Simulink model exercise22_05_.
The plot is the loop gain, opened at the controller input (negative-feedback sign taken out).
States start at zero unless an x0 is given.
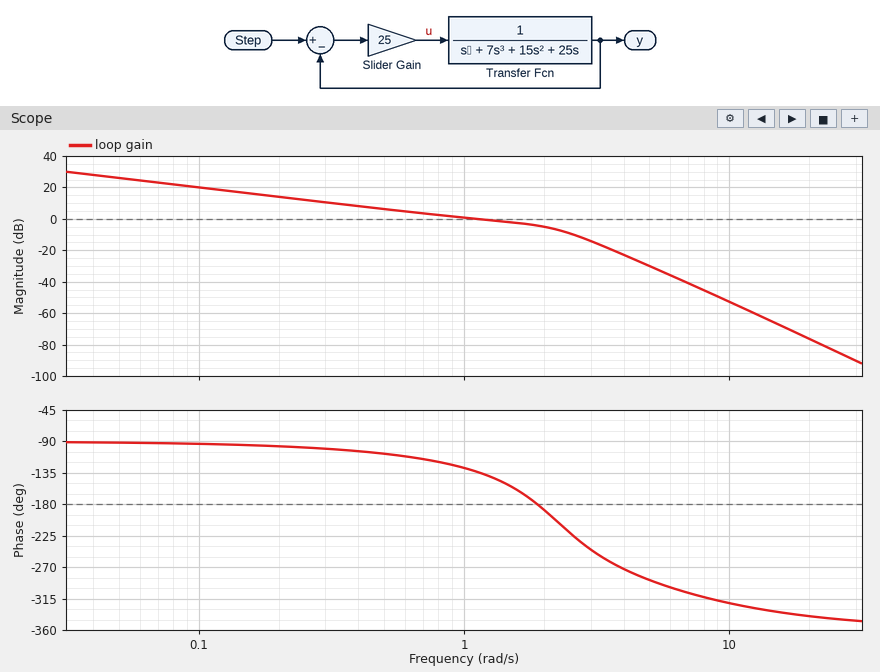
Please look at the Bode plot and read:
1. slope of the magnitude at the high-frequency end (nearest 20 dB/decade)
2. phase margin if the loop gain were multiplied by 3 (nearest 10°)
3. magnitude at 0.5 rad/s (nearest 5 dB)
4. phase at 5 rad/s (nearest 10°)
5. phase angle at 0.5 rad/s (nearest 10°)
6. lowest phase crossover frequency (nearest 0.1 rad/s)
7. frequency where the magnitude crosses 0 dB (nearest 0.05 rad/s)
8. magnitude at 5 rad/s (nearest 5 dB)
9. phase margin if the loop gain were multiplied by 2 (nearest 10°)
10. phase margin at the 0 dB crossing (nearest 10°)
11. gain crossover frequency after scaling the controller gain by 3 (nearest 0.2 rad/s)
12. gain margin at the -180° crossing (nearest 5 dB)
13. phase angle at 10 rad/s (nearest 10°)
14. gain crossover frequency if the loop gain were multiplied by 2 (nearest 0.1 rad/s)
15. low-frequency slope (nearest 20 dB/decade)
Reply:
-80 dB/decade
-40°
5 dB
-290°
-110°
1.9 rad/s
1.10 rad/s
-30 dB
-20°
50°
2.6 rad/s
5 dB
-320°
2.1 rad/s
-20 dB/decade
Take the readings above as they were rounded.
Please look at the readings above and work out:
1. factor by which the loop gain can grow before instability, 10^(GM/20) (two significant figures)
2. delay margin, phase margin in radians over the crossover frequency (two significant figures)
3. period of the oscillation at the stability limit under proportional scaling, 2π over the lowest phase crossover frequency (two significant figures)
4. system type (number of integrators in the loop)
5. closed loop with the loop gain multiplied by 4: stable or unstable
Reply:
1.8
0.79 s
3.3 s
1
unstable
